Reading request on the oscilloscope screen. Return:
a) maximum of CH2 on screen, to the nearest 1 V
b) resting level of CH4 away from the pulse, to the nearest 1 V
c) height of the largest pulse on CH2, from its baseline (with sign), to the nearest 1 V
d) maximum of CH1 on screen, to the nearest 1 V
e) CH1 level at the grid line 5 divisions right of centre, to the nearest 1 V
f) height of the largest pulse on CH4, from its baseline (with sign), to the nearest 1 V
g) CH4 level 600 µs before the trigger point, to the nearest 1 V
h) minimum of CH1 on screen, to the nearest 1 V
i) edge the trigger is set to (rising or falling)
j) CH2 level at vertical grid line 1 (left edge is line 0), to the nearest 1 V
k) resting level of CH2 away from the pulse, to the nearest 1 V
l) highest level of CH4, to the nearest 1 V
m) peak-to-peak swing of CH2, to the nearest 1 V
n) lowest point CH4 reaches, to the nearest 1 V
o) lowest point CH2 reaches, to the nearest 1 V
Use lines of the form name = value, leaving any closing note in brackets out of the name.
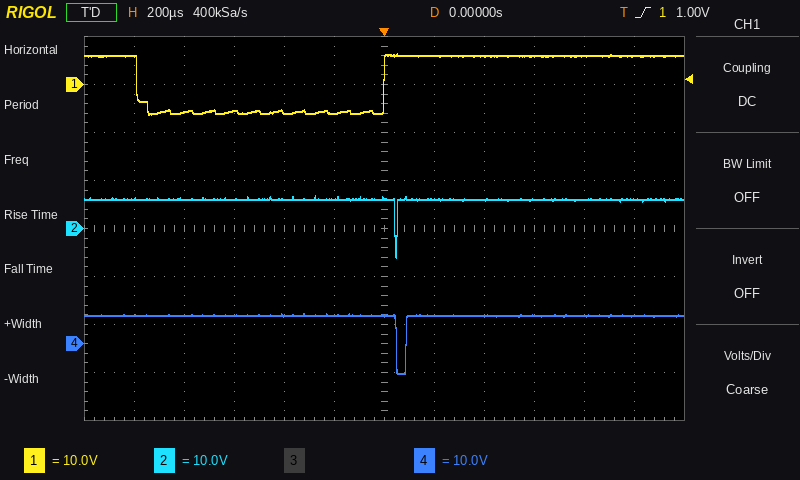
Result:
maximum of CH2 on screen, to the nearest 1 V = 7 V
resting level of CH4 away from the pulse, to the nearest 1 V = 6 V
height of the largest pulse on CH2, from its baseline (with sign), to the nearest 1 V = -12 V
maximum of CH1 on screen, to the nearest 1 V = 6 V
CH1 level at the grid line 5 divisions right of centre, to the nearest 1 V = 6 V
height of the largest pulse on CH4, from its baseline (with sign), to the nearest 1 V = -12 V
CH4 level 600 µs before the trigger point, to the nearest 1 V = 6 V
minimum of CH1 on screen, to the nearest 1 V = -6 V
edge the trigger is set to = rising
CH2 level at vertical grid line 1 (left edge is line 0), to the nearest 1 V = 6 V
resting level of CH2 away from the pulse, to the nearest 1 V = 6 V
highest level of CH4, to the nearest 1 V = 6 V
peak-to-peak swing of CH2, to the nearest 1 V = 13 V
lowest point CH4 reaches, to the nearest 1 V = -6 V
lowest point CH2 reaches, to the nearest 1 V = -6 V
